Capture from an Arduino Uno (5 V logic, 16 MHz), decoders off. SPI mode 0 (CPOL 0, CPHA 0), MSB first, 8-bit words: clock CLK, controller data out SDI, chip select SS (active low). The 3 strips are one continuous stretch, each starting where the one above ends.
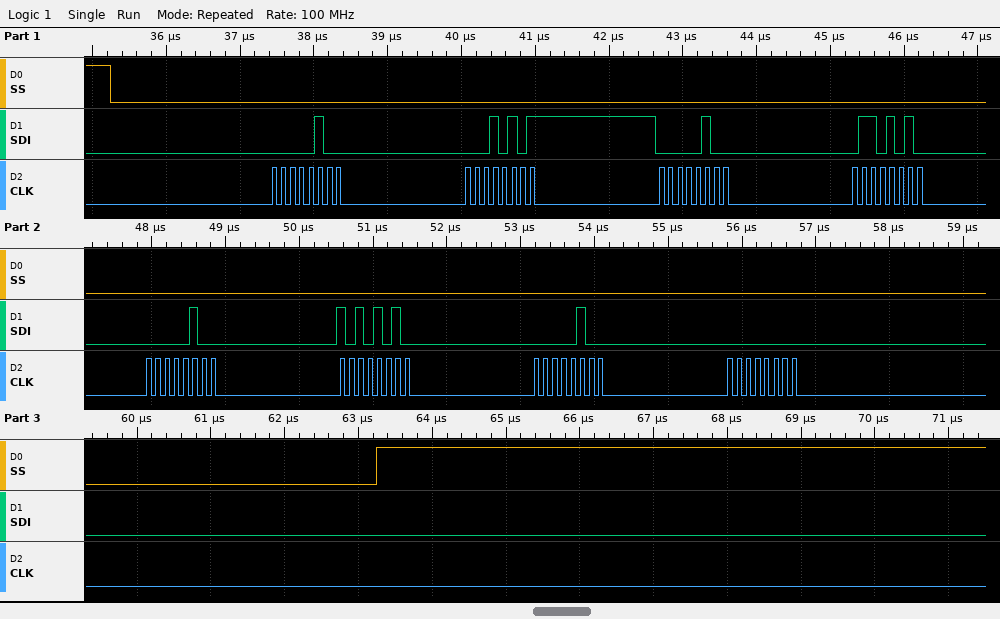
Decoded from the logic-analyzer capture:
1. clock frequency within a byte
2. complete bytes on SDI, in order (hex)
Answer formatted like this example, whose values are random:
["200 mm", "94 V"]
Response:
["8 MHz", "04 15 04 6A 04 AA 04 00"]
